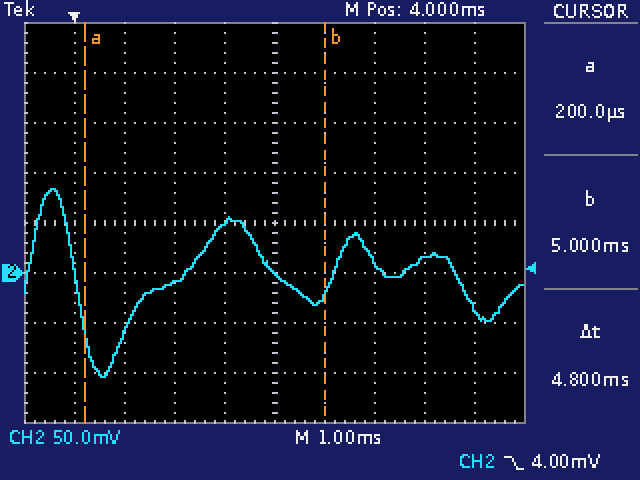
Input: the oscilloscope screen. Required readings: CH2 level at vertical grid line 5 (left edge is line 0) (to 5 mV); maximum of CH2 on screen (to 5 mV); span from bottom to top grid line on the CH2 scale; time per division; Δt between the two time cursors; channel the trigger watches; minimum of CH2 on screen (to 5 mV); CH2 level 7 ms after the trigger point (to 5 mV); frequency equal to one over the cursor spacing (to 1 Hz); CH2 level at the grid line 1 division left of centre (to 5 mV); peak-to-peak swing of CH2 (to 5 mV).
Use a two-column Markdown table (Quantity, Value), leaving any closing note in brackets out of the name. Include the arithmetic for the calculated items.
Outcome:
| Quantity | Value |
|---|---|
| CH2 level at vertical grid line 5 (left edge is line 0) | 0 mV |
| maximum of CH2 on screen | 85 mV |
| span from bottom to top grid line on the CH2 scale | 400 mV |
| time per division | 1 ms |
| Δt between the two time cursors | 4.8 ms |
| channel the trigger watches | CH2 |
| minimum of CH2 on screen | -105 mV |
| CH2 level 7 ms after the trigger point | 15 mV |
| frequency equal to one over the cursor spacing | 1 / 4.8 ms ≈ 208 Hz |
| CH2 level at the grid line 1 division left of centre | 50 mV |
| peak-to-peak swing of CH2 | 85 mV − (-105 mV) = 190 mV |
